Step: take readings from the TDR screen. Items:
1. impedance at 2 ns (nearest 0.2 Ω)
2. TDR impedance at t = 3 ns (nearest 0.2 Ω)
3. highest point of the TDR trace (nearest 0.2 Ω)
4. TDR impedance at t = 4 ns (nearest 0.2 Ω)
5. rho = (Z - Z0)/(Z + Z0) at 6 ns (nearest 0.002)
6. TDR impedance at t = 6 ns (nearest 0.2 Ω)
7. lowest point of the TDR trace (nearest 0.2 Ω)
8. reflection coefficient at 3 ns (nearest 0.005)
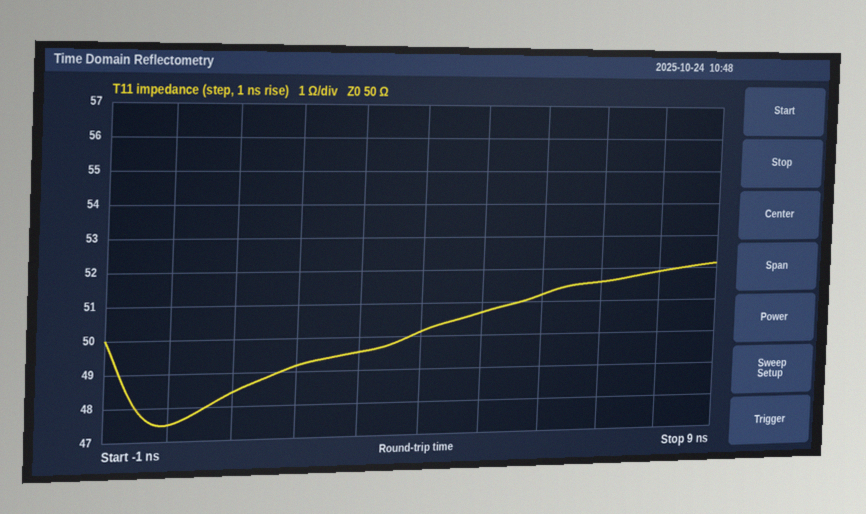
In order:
49.2 Ω
49.6 Ω
52.2 Ω
50.2 Ω
+0.012
51.2 Ω
47.4 Ω
-0.005
